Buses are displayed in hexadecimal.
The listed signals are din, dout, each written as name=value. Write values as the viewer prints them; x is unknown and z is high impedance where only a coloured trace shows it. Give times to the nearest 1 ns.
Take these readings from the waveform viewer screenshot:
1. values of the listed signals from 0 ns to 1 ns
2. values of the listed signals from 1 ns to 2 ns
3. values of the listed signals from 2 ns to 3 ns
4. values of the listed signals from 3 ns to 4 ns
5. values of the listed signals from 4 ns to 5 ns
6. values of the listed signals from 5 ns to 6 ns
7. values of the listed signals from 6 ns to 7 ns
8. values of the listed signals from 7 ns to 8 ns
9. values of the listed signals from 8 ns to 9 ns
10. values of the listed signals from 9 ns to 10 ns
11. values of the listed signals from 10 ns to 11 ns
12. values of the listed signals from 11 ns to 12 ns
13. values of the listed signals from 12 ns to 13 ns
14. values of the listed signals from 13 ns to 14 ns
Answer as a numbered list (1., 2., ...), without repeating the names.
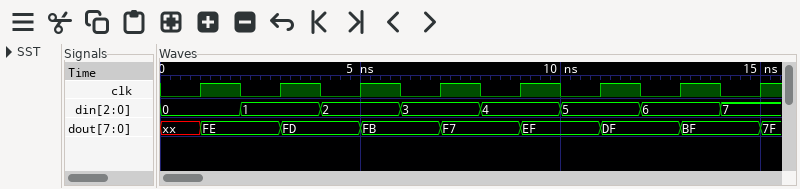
1. din=0, dout=xx
2. din=0, dout=FE
3. din=1, dout=FE
4. din=1, dout=FD
5. din=2, dout=FD
6. din=2, dout=FB
7. din=3, dout=FB
8. din=3, dout=F7
9. din=4, dout=F7
10. din=4, dout=EF
11. din=5, dout=EF
12. din=5, dout=DF
13. din=6, dout=DF
14. din=6, dout=BF
